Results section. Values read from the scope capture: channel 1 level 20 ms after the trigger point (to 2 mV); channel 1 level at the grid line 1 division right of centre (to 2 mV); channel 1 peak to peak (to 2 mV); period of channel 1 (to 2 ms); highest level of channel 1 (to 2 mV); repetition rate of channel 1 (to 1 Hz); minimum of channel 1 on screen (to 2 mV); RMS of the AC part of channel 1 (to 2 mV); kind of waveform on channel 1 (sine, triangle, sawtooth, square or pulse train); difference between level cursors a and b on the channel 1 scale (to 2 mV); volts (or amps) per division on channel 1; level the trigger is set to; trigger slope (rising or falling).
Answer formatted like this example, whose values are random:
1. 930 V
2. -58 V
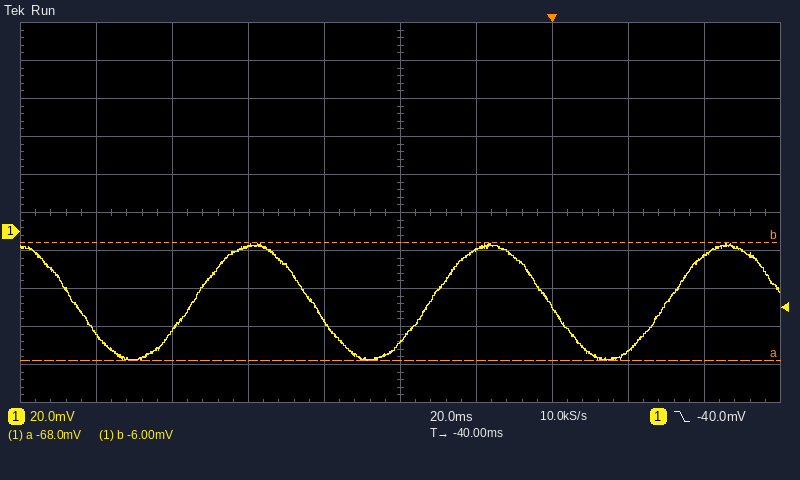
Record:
1. -62 mV
2. -10 mV
3. 62 mV
4. 62 ms
5. -6 mV
6. 16 Hz
7. -68 mV
8. 22 mV
9. sine
10. 62 mV
11. 20 mV
12. -40.0 mV
13. falling
